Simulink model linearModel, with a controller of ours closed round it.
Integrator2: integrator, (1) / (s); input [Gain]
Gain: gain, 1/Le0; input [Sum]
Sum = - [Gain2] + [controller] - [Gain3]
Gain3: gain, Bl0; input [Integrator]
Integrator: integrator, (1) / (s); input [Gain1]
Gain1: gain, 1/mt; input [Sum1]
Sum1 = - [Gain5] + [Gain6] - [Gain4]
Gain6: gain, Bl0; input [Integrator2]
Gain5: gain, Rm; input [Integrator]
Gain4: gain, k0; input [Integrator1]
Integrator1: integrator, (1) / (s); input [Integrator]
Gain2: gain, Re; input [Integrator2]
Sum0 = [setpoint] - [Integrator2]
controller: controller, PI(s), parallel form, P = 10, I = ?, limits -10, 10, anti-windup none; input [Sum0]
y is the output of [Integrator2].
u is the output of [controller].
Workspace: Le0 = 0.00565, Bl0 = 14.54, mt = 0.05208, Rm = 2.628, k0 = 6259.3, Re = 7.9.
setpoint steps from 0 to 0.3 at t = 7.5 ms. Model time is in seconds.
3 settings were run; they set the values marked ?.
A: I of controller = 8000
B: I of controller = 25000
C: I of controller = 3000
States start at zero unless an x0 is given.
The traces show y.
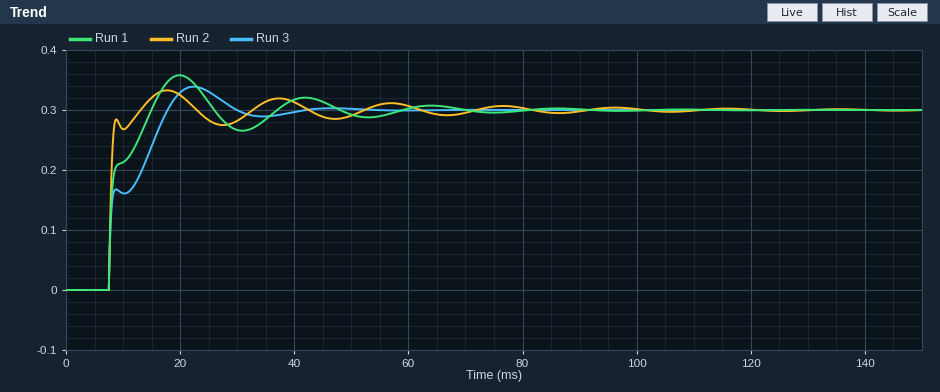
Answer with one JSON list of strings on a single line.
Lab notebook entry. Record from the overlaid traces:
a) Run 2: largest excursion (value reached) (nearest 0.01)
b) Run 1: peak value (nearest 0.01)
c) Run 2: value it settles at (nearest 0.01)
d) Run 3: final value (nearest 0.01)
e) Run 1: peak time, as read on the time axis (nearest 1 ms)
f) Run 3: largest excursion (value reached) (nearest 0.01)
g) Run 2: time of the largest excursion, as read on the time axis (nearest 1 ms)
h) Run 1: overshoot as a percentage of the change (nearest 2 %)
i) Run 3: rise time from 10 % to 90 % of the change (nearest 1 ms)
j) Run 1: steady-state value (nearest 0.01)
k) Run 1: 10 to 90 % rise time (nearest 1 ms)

["0.33", "0.36", "0.30", "0.30", "20 ms", "0.34", "18 ms", "20 %", "9 ms", "0.30", "6 ms"]
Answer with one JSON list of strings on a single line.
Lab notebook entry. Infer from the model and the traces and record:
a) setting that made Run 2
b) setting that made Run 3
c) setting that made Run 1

["B", "C", "A"]
